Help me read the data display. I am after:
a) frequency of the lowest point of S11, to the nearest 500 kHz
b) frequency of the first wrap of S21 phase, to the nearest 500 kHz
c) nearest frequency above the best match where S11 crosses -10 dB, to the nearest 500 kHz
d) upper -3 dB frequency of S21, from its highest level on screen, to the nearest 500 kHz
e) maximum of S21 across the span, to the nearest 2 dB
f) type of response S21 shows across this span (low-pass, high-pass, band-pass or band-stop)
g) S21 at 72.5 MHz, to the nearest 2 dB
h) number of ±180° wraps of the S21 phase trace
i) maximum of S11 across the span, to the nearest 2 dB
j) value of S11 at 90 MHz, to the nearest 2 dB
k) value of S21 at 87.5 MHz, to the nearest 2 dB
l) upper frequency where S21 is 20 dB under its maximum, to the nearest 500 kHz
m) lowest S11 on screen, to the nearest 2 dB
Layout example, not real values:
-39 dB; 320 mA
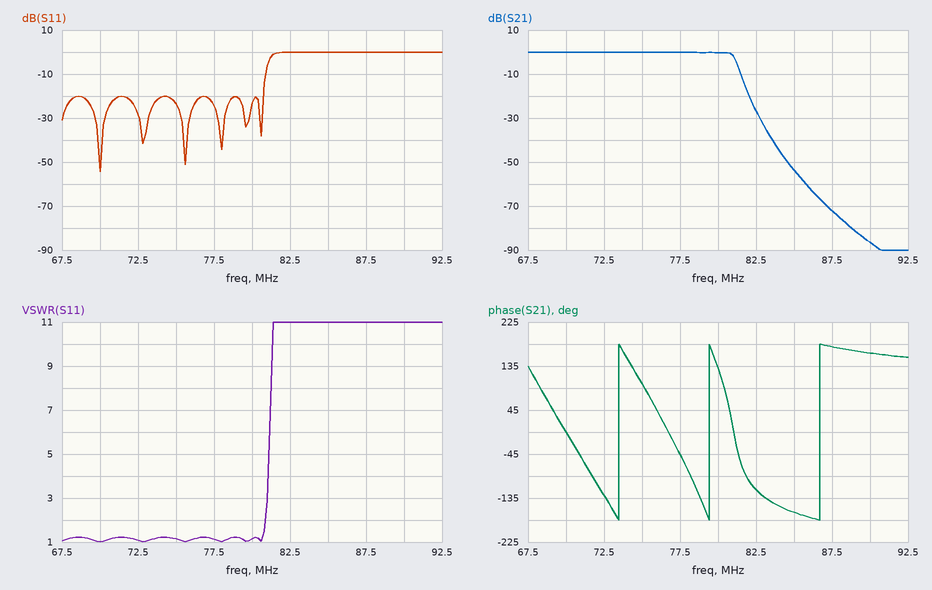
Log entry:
70.0 MHz; 73.5 MHz; 81.0 MHz; 81.0 MHz; 0 dB; low-pass; 0 dB; 3; 0 dB; 0 dB; -72 dB; 82.0 MHz; -54 dB
